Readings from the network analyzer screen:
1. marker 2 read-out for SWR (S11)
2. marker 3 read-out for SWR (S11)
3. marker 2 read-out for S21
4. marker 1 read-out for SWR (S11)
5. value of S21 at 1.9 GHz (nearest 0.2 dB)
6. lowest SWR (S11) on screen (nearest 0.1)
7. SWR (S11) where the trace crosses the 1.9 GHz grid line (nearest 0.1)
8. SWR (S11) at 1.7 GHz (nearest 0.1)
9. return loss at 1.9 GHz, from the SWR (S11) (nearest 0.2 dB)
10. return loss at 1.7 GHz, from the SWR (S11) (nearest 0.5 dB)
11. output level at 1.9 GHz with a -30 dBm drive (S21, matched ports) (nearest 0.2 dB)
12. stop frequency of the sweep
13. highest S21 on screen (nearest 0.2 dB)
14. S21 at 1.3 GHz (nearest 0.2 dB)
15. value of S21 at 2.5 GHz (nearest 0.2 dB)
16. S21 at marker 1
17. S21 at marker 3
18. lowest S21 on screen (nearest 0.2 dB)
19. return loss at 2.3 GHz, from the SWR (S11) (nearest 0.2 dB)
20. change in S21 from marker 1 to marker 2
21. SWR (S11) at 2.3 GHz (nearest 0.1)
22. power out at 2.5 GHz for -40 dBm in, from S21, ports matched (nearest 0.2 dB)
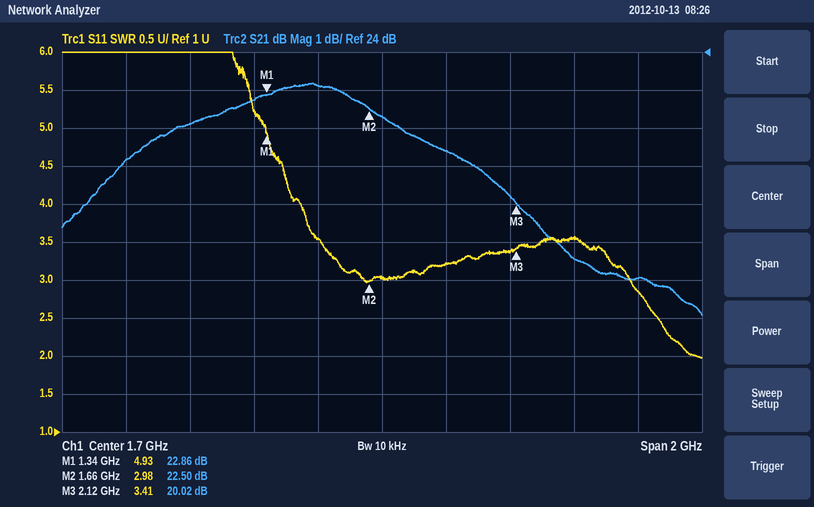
2.98
3.41
22.50 dB
4.93
21.4 dB
2.0
3.2
3.0
5.6 dB
6.0 dB
-8.6 dBm
2.7 GHz
23.2 dB
22.8 dB
18.0 dB
22.86 dB
20.02 dB
17.0 dB
5.0 dB
-0.36 dB
3.6
-22.0 dBm
